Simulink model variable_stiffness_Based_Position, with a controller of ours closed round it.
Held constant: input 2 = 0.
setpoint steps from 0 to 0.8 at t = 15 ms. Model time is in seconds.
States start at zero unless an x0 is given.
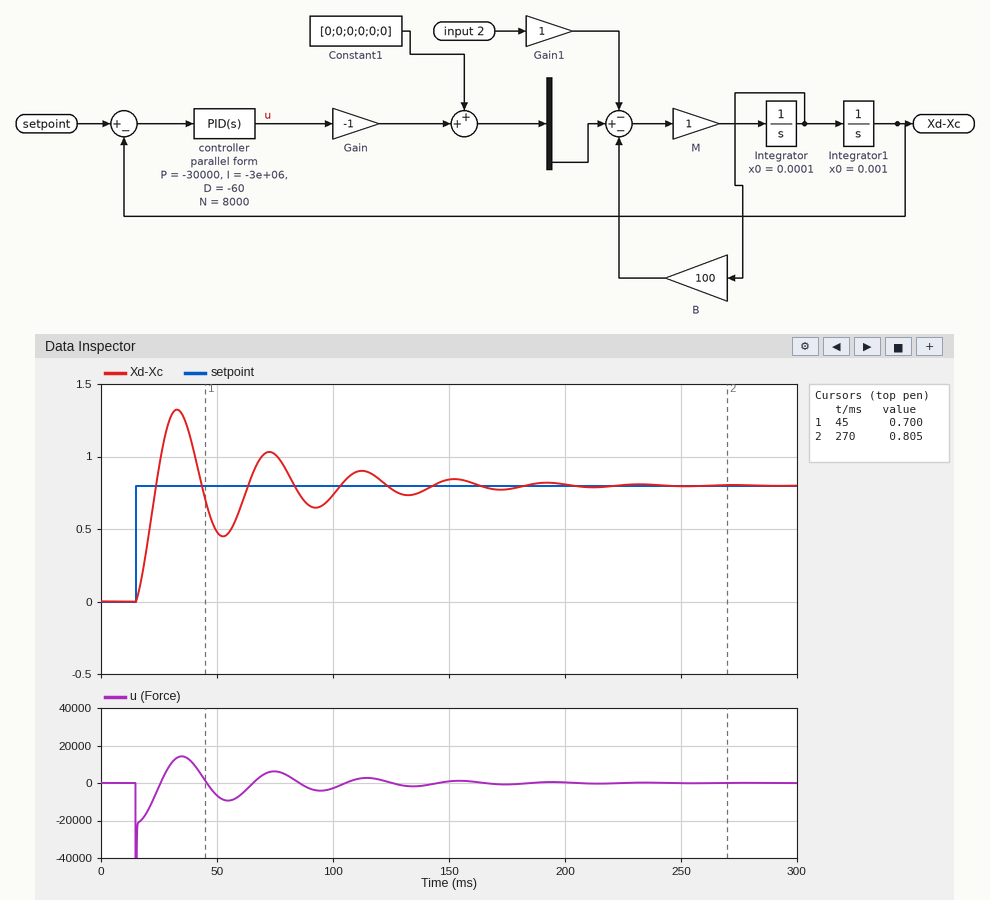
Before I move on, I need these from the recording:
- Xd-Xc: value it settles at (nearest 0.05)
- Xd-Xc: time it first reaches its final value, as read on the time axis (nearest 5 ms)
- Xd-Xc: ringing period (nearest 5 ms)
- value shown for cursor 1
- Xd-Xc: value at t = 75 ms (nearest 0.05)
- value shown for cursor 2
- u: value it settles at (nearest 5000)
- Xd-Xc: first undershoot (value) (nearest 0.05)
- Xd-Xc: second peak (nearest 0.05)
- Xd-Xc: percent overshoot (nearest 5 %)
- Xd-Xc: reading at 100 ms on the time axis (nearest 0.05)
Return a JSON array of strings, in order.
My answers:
["0.80", "25 ms", "40 ms", "0.700", "1.00", "0.805", "0", "0.45", "1.05", "65 %", "0.75"]
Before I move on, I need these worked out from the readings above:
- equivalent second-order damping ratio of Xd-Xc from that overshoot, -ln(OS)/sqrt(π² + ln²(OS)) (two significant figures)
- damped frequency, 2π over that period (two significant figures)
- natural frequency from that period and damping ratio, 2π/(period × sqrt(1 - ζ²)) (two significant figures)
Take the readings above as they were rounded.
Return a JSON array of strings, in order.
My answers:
["0.14", "0.16 rad/ms", "0.16 rad/ms"]
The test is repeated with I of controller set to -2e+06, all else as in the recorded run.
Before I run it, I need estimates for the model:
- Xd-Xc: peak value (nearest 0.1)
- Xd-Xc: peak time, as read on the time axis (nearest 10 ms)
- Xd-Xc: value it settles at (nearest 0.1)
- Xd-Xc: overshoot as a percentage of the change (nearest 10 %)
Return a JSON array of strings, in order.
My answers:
["1.2", "30 ms", "0.8", "50 %"]
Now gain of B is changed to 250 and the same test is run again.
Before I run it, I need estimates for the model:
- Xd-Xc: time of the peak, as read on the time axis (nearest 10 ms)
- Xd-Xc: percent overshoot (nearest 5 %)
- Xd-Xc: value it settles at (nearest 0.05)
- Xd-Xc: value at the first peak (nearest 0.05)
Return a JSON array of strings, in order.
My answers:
["40 ms", "45 %", "0.80", "1.15"]
